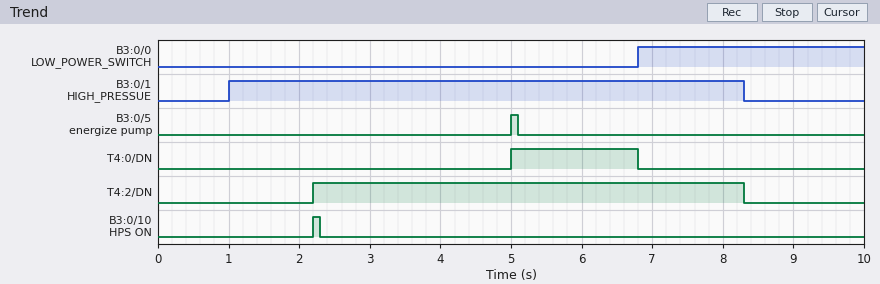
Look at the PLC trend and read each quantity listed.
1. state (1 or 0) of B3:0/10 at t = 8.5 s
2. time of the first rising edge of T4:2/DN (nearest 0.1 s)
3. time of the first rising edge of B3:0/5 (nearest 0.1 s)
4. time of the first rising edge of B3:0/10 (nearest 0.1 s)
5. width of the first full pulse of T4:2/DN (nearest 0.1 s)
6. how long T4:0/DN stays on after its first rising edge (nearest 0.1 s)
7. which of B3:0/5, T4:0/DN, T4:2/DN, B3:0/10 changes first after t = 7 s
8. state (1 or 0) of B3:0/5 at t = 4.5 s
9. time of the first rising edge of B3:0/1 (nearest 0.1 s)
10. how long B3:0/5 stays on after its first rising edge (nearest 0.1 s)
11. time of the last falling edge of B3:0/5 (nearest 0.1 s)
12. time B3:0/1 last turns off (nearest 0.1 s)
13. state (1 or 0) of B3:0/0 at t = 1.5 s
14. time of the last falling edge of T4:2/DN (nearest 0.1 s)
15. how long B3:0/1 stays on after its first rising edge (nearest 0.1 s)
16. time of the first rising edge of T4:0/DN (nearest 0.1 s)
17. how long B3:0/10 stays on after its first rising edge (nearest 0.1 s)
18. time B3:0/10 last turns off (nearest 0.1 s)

0
2.2 s
5.0 s
2.2 s
6.1 s
1.8 s
T4:2/DN
0
1.0 s
0.1 s
5.1 s
8.3 s
0
8.3 s
7.3 s
5.0 s
0.1 s
2.3 s
